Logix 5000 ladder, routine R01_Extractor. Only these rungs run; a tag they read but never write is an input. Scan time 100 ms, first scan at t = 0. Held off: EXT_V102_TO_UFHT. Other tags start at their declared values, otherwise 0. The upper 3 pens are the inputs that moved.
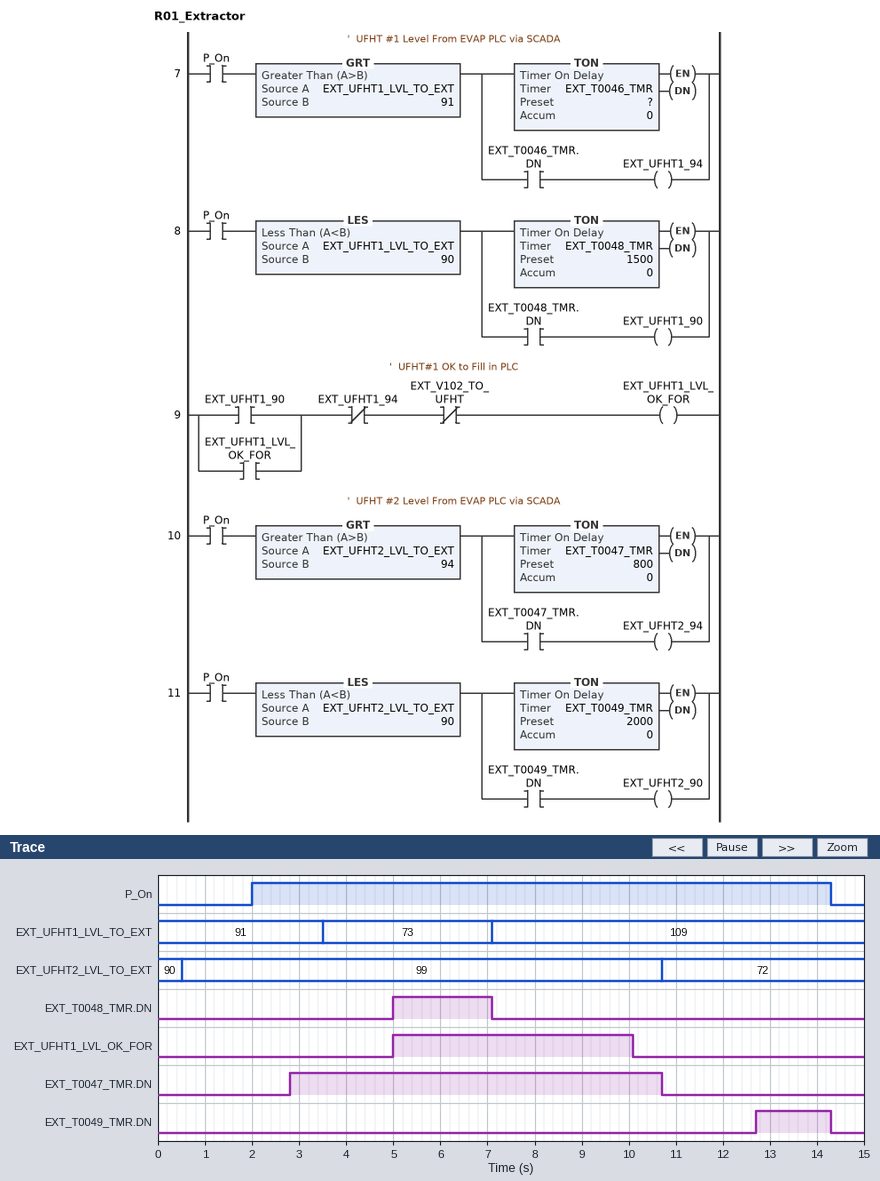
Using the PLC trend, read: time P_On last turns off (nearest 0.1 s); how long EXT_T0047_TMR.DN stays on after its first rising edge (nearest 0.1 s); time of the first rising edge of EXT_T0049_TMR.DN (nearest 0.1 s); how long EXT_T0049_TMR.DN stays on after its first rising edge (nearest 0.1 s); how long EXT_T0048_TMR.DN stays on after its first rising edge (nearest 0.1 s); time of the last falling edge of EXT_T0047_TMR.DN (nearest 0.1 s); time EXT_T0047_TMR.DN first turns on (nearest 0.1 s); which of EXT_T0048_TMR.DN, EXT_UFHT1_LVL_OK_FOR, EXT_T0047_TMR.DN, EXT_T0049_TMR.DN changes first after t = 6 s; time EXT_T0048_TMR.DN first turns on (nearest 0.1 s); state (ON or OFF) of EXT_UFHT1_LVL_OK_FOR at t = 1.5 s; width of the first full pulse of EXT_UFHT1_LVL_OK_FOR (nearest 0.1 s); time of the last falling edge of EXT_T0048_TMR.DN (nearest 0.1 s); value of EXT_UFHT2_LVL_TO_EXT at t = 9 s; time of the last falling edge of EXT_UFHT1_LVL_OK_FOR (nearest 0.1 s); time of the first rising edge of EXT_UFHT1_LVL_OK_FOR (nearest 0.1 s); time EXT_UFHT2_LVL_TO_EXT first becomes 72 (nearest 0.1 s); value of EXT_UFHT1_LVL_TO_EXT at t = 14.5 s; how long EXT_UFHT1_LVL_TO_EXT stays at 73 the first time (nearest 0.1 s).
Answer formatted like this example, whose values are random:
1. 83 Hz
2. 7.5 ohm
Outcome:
1. 14.3 s
2. 7.9 s
3. 12.7 s
4. 1.6 s
5. 2.1 s
6. 10.7 s
7. 2.8 s
8. EXT_T0048_TMR.DN
9. 5.0 s
10. OFF
11. 5.1 s
12. 7.1 s
13. 99
14. 10.1 s
15. 5.0 s
16. 10.7 s
17. 109
18. 3.6 s
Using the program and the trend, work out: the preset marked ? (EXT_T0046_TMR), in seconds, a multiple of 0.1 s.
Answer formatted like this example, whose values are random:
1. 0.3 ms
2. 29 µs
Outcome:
1. 3.0 s
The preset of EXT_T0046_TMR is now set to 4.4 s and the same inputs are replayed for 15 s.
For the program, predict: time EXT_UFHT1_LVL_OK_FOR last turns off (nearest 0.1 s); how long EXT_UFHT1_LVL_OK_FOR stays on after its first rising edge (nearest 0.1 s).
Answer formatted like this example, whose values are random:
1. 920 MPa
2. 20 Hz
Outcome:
1. 11.5 s
2. 6.5 s
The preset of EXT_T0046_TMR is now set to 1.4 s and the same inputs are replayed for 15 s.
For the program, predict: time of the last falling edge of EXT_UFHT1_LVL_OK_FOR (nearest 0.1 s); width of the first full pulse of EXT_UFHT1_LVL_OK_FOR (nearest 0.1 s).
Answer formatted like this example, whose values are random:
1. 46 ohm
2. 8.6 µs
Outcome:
1. 8.5 s
2. 3.5 s
